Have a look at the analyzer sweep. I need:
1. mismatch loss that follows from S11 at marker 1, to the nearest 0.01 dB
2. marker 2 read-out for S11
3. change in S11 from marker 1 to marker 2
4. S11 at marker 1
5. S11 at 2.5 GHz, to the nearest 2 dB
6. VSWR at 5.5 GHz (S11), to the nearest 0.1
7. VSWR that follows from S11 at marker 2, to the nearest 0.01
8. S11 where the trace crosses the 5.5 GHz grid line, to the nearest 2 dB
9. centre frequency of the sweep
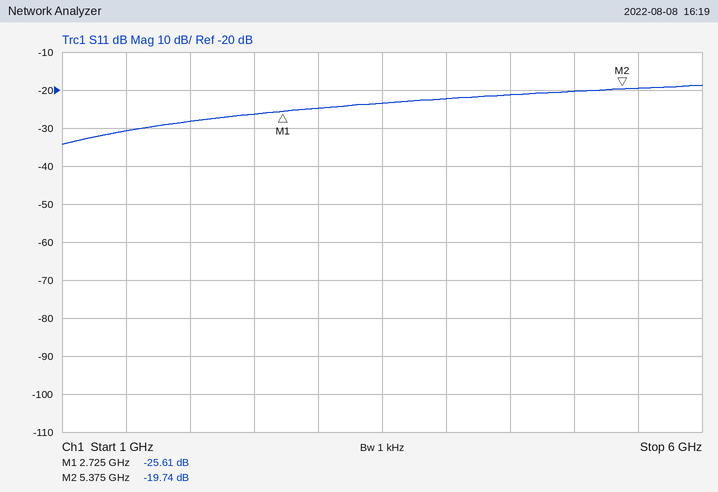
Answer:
0.01 dB
-19.74 dB
5.87 dB
-25.61 dB
-26 dB
1.2
1.23
-20 dB
3.5 GHz
